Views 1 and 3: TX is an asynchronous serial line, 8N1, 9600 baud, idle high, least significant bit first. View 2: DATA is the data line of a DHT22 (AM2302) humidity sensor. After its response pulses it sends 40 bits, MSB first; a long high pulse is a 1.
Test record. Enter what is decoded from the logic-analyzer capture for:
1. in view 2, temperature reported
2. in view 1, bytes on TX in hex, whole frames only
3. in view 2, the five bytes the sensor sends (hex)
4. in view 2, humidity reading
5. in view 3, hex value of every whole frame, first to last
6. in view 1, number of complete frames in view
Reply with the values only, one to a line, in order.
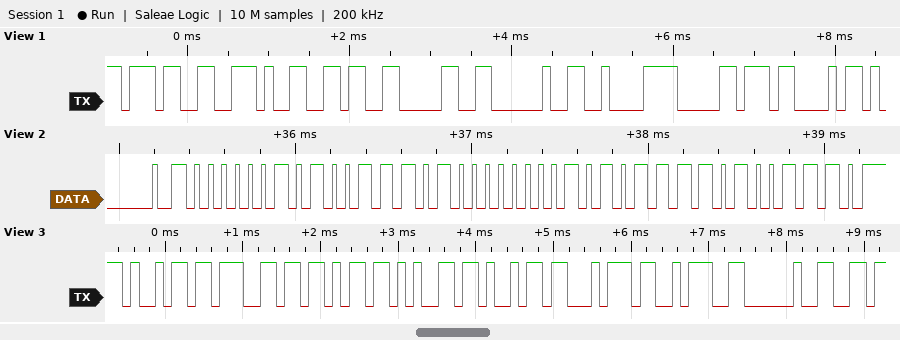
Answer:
17.5 °C
37 2E 36 30 20 C2 B0 43
02 9D 00 AF 4E
66.9 %
69 67 6B 65 69 74 3A 20
8
